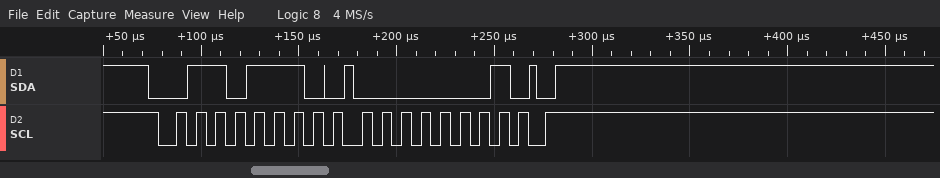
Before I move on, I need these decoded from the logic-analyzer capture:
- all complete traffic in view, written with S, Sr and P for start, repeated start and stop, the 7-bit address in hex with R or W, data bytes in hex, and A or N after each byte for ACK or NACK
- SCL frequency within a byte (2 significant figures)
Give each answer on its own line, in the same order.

S 37W A 01 A P
100 kHz
